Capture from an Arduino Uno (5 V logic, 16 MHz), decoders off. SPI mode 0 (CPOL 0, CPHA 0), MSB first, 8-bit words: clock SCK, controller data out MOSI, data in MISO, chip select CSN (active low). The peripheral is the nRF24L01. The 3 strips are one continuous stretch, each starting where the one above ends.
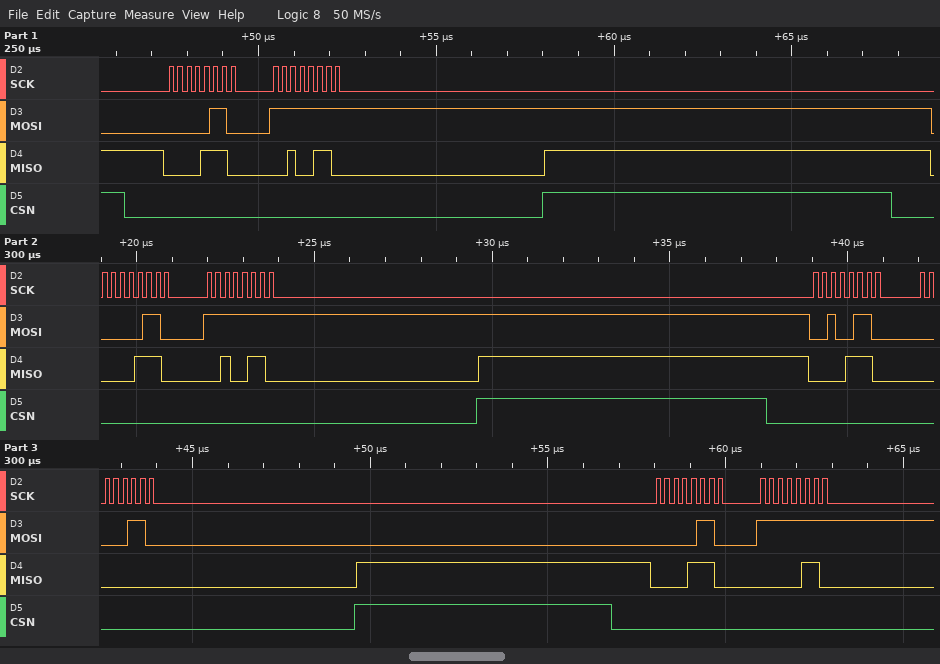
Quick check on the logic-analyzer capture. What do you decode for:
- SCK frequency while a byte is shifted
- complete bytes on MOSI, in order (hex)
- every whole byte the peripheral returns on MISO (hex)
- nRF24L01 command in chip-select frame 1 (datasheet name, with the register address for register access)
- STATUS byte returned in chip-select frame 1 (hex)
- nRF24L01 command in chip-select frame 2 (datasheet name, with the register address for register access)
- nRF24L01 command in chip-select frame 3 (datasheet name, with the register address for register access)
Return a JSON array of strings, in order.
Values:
["4 MHz", "06 FF 06 FF 26 06 06 FF", "0E 26 0E 26 0E 00 0E 06", "R_REGISTER 0x06", "0x0E", "R_REGISTER 0x06", "W_REGISTER 0x06"]
